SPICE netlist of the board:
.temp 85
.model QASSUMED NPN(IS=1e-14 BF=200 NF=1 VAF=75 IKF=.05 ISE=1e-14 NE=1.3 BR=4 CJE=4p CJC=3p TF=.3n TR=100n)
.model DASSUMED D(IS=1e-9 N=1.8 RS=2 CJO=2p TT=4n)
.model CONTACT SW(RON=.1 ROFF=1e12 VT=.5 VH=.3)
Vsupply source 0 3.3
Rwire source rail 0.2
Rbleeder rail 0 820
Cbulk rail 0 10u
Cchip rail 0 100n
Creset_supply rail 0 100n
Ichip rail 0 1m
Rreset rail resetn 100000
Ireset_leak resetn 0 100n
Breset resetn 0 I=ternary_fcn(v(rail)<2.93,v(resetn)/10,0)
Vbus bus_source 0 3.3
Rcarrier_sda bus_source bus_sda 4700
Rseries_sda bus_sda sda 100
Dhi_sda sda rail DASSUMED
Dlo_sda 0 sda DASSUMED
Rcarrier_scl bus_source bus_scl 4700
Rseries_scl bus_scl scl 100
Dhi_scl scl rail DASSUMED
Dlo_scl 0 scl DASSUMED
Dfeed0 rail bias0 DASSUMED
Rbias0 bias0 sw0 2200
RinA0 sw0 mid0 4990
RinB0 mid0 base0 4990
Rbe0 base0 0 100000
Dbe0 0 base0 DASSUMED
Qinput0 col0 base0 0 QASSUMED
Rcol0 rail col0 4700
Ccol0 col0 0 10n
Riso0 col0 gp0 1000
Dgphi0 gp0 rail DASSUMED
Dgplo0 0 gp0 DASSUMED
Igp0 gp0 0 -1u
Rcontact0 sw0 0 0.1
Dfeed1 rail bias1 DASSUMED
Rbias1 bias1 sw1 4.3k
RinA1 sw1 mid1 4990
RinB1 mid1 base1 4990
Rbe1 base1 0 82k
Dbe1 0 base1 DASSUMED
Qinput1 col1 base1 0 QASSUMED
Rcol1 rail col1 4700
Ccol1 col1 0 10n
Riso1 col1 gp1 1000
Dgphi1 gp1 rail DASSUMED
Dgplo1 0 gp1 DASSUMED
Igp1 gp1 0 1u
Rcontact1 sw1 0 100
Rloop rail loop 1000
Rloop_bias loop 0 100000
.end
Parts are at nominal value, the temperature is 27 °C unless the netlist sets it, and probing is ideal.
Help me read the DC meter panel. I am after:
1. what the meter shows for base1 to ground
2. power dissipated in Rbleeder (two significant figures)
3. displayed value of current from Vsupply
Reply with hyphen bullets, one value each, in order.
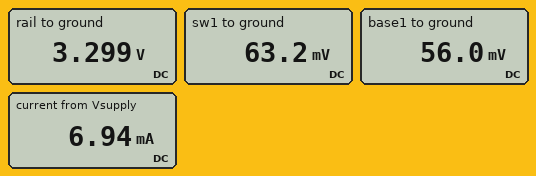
- 56.0 mV
- 13 mW
- 6.94 mA
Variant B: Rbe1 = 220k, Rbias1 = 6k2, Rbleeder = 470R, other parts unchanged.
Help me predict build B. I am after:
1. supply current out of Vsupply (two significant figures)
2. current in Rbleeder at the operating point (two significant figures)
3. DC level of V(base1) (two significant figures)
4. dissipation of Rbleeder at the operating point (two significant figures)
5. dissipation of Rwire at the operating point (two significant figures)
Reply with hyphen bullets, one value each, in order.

- 9.7 mA
- 7.0 mA
- 42 mV
- 23 mW
- 19 µW
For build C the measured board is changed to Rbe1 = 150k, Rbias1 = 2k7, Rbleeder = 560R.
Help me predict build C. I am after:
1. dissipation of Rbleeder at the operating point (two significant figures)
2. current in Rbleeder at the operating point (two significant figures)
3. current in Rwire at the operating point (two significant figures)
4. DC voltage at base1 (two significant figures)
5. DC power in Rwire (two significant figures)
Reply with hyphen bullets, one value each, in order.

- 19 mW
- 5.9 mA
- 9.2 mA
- 92 mV
- 17 µW
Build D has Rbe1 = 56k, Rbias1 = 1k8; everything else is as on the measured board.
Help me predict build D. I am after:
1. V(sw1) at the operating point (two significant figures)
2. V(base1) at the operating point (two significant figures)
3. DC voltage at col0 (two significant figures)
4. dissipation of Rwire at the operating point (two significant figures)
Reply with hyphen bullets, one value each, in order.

- 140 mV
- 120 mV
- 3.3 V
- 12 µW
